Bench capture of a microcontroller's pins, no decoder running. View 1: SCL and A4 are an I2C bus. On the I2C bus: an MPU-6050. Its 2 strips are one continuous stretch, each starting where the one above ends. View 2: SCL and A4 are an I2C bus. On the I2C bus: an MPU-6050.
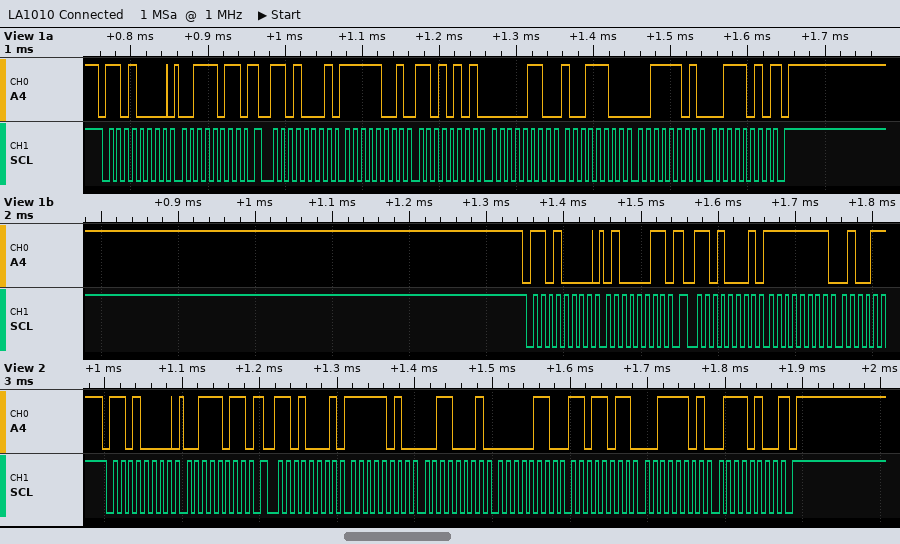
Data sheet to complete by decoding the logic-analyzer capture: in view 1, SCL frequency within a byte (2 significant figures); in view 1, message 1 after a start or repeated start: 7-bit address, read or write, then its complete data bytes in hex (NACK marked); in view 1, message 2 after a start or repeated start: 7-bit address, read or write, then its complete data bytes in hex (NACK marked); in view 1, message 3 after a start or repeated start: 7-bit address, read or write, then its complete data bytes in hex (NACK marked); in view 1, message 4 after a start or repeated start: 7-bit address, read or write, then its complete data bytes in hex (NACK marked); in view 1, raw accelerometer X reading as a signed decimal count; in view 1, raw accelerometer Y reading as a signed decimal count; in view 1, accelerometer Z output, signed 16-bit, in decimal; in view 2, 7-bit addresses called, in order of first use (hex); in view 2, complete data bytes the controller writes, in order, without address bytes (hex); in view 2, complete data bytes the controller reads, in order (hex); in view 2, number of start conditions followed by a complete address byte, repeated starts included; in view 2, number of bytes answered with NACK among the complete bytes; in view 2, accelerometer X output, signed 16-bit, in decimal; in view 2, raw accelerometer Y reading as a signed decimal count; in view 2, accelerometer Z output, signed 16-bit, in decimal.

100 kHz
0x68 write: 3B
0x68 read: F9 D5 06 9C 3D 3A NACK
0x68 write: 43
0x68 read: FF
-1579
1692
15674
0x68
3B
FA 31 06 DB 3D 74
2
1
-1487
1755
15732
